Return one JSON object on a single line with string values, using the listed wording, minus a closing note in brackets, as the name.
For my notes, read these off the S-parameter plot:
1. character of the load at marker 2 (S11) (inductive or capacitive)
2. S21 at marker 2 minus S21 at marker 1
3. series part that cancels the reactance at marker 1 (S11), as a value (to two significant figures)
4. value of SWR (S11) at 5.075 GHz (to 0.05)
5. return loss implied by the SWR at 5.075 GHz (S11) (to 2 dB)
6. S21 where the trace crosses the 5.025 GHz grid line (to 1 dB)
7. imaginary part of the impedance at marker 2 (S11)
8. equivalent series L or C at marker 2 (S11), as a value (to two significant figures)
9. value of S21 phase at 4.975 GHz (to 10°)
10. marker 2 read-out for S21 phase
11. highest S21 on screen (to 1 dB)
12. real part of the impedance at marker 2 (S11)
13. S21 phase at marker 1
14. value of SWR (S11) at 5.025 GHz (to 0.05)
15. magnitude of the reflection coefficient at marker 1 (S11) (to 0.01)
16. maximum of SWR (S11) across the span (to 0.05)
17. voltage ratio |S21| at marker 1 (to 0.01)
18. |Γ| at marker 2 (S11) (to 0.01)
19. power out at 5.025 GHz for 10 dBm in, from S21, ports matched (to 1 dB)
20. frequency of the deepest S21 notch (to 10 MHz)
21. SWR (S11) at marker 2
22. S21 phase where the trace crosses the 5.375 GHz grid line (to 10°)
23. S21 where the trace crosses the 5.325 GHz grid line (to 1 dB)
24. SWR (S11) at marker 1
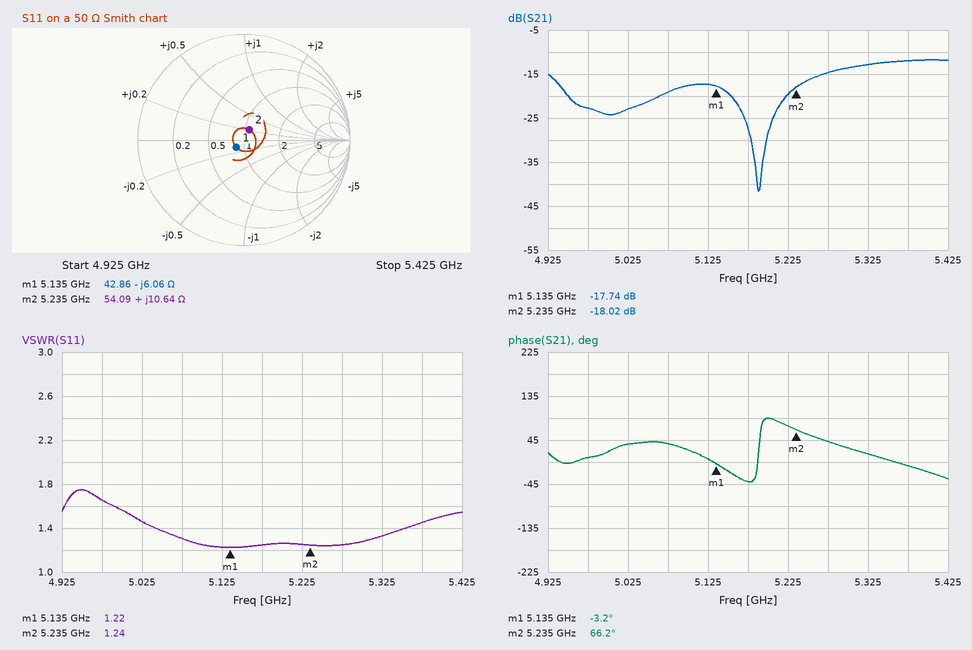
{"character of the load at marker 2 (S11)": "inductive", "S21 at marker 2 minus S21 at marker 1": "-0.28 dB", "series part that cancels the reactance at marker 1 (S11), as a value": "190 pH", "value of SWR (S11) at 5.075 GHz": "1.30", "return loss implied by the SWR at 5.075 GHz (S11)": "18 dB", "S21 where the trace crosses the 5.025 GHz grid line": "-23 dB", "imaginary part of the impedance at marker 2": "+10.64 Ω", "equivalent series L or C at marker 2 (S11), as a value": "320 pH", "value of S21 phase at 4.975 GHz": "10°", "marker 2 read-out for S21 phase": "66.2°", "highest S21 on screen": "-12 dB", "real part of the impedance at marker 2": "54.09 Ω", "S21 phase at marker 1": "-3.2°", "value of SWR (S11) at 5.025 GHz": "1.45", "magnitude of the reflection coefficient at marker 1 (S11)": "0.10", "maximum of SWR (S11) across the span": "1.75", "voltage ratio |S21| at marker 1": "0.13", "|Γ| at marker 2 (S11)": "0.11", "power out at 5.025 GHz for 10 dBm in, from S21, ports matched": "-13 dBm", "frequency of the deepest S21 notch": "5.19 GHz", "SWR (S11) at marker 2": "1.24", "S21 phase where the trace crosses the 5.375 GHz grid line": "-10°", "S21 where the trace crosses the 5.325 GHz grid line": "-13 dB", "SWR (S11) at marker 1": "1.22"}
